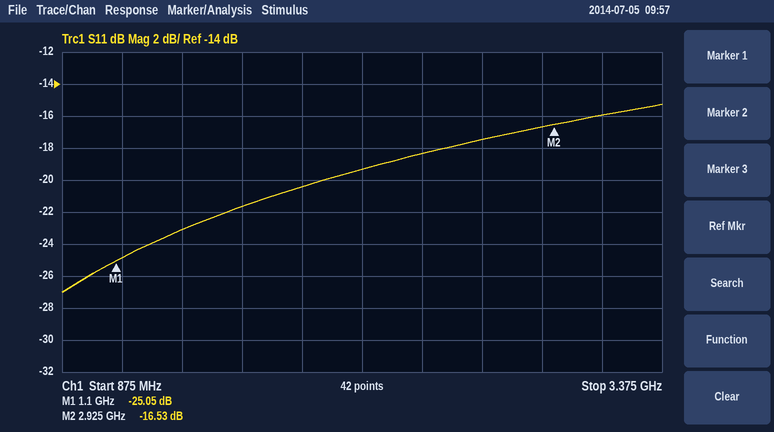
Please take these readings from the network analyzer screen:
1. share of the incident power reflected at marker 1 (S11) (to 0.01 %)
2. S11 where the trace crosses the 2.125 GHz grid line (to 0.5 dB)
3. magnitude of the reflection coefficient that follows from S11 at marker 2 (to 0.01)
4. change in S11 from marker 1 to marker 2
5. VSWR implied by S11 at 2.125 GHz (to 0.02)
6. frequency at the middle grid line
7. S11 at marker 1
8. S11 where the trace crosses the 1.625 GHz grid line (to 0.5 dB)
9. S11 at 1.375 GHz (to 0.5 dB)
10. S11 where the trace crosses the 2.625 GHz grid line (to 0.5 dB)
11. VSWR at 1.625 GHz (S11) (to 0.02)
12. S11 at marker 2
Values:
0.31 %
-19.5 dB
0.15
8.52 dB
1.24
2.125 GHz
-25.05 dB
-21.5 dB
-23.0 dB
-17.5 dB
1.18
-16.53 dB
